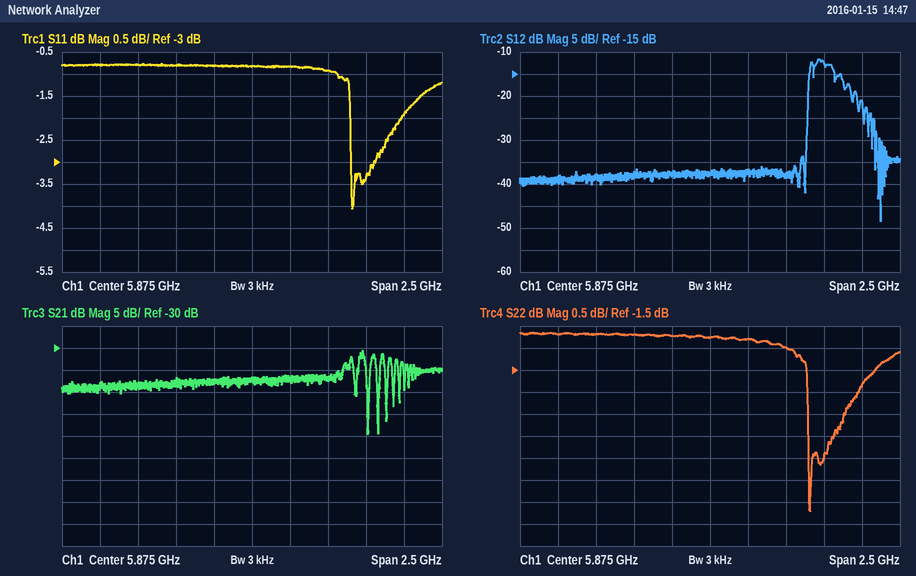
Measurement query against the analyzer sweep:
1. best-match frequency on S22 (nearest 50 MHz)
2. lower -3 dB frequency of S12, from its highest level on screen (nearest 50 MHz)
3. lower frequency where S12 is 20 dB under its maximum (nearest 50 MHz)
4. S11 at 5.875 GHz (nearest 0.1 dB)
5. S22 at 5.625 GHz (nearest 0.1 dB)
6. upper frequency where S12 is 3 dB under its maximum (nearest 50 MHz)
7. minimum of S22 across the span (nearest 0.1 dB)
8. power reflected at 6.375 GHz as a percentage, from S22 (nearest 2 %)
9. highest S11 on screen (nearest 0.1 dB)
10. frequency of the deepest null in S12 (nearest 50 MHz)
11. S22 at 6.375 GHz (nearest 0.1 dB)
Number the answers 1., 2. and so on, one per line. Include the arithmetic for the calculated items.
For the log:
1. 6.55 GHz
2. 6.55 GHz
3. 6.50 GHz
4. -0.8 dB
5. -0.7 dB
6. 6.70 GHz
7. -4.7 dB
8. 10^(-1/10) ≈ 79.4 %, so 80 % to the nearest 2 %
9. -0.8 dB
10. 7.00 GHz
11. -1.0 dB
